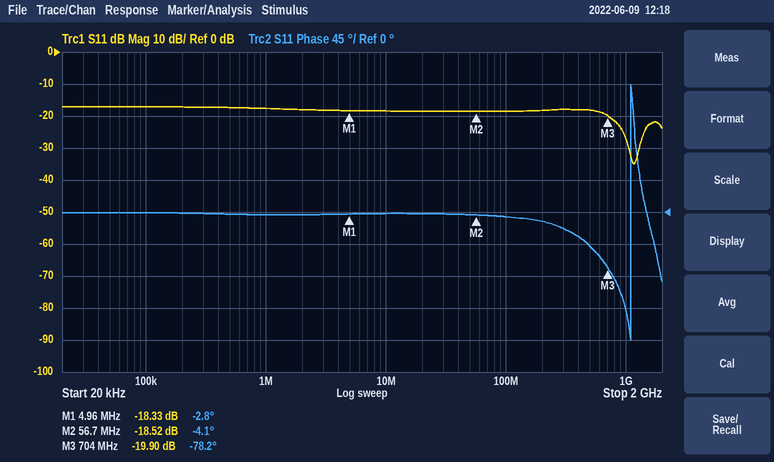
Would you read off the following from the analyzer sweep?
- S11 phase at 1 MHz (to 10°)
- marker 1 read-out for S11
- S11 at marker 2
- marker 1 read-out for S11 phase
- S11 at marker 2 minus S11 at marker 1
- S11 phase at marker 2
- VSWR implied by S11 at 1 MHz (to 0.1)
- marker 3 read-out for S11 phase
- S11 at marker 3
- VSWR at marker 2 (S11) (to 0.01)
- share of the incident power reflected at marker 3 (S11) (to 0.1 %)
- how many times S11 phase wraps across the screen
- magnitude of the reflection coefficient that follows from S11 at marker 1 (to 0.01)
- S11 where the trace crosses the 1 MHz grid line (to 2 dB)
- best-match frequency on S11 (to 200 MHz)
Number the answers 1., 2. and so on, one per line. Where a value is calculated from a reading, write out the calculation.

1. 0°
2. -18.33 dB
3. -18.52 dB
4. -2.8°
5. -18.52 − (-18.33) = -0.19 dB
6. -4.1°
7. |Γ| = 10^(-18/20) = 0.1259; VSWR = (1 + 0.1259)/(1 − 0.1259) ≈ 1.3
8. -78.2°
9. -19.90 dB
10. (1 + 0.1186)/(1 − 0.1186) ≈ 1.27
11. 10^(-19.9/10) ≈ 1.0 %
12. 1
13. 10^(-18.33/20) ≈ 0.12
14. -18 dB
15. 1.2 GHz
